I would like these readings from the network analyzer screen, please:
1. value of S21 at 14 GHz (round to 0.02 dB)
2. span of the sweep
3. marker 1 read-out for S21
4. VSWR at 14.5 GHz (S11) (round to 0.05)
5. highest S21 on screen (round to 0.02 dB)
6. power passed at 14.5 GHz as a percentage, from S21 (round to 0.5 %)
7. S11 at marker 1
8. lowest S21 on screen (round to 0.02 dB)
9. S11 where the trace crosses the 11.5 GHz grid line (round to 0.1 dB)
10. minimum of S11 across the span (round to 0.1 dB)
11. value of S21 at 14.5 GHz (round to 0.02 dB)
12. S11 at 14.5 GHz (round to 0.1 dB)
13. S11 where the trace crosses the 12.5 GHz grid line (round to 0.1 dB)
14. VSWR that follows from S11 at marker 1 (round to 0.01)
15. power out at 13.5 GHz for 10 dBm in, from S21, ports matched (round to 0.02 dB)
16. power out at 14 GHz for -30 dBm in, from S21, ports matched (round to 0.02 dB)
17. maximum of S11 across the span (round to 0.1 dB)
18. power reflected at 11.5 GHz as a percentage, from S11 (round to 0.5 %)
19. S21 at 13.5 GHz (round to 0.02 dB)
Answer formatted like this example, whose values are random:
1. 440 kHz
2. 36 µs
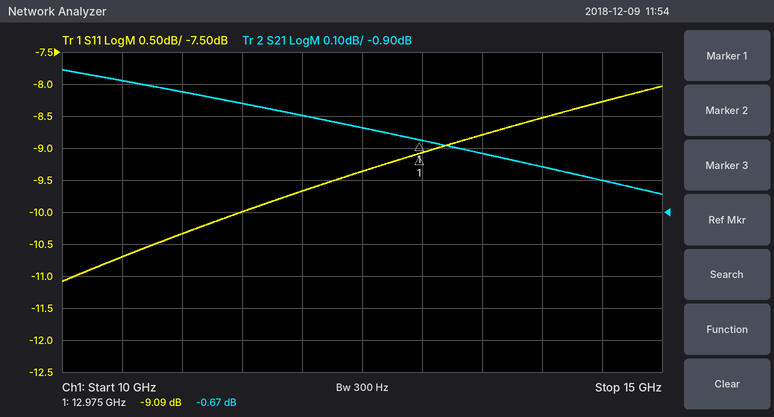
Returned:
1. -0.76 dB
2. 5 GHz
3. -0.67 dB
4. 2.25
5. -0.46 dB
6. 83.0 %
7. -9.09 dB
8. -0.84 dB
9. -10.0 dB
10. -11.1 dB
11. -0.80 dB
12. -8.3 dB
13. -9.4 dB
14. 2.08
15. 9.28 dBm
16. -30.76 dBm
17. -8.0 dB
18. 10.0 %
19. -0.72 dB
